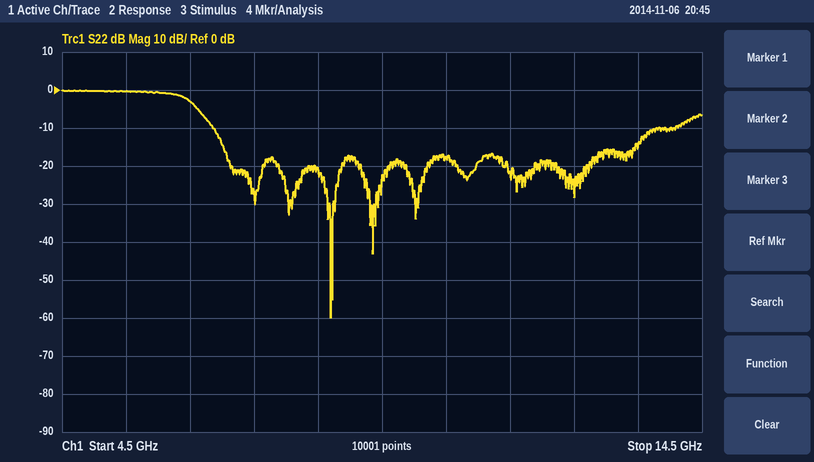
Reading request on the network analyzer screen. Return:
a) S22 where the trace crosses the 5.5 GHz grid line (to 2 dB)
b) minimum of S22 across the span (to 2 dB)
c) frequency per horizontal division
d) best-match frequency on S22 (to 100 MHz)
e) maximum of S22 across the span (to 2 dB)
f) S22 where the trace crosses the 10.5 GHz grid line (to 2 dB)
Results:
0 dB
-60 dB
1 GHz
8.7 GHz
0 dB
-18 dB
